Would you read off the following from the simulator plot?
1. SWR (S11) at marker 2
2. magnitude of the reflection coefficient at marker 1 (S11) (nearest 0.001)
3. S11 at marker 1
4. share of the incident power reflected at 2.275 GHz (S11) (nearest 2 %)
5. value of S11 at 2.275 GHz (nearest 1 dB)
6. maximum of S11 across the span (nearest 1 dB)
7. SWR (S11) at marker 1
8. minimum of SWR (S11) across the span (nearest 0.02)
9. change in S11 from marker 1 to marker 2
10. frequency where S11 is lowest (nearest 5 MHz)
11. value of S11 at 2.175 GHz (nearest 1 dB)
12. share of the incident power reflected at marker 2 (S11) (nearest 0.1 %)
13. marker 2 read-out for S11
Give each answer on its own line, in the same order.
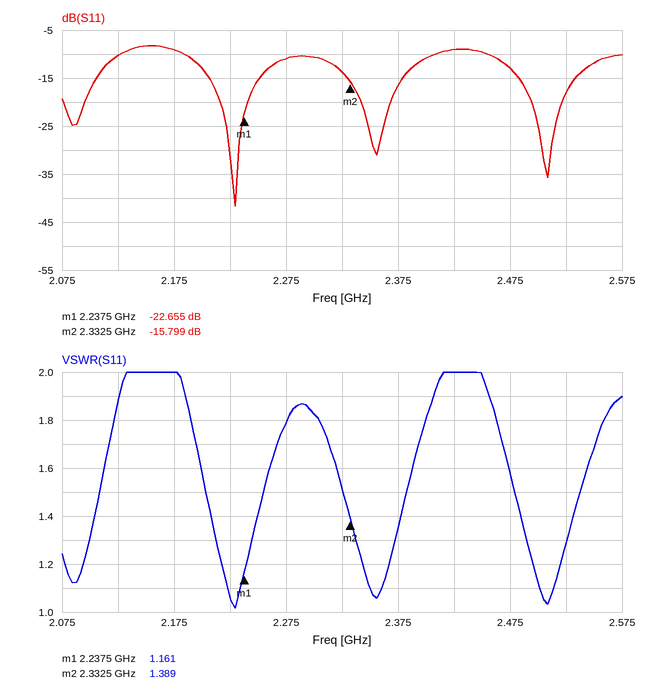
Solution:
1.389
0.074
-22.655 dB
8 %
-11 dB
-8 dB
1.161
1.02
6.856 dB
2.230 GHz
-9 dB
2.6 %
-15.799 dB
